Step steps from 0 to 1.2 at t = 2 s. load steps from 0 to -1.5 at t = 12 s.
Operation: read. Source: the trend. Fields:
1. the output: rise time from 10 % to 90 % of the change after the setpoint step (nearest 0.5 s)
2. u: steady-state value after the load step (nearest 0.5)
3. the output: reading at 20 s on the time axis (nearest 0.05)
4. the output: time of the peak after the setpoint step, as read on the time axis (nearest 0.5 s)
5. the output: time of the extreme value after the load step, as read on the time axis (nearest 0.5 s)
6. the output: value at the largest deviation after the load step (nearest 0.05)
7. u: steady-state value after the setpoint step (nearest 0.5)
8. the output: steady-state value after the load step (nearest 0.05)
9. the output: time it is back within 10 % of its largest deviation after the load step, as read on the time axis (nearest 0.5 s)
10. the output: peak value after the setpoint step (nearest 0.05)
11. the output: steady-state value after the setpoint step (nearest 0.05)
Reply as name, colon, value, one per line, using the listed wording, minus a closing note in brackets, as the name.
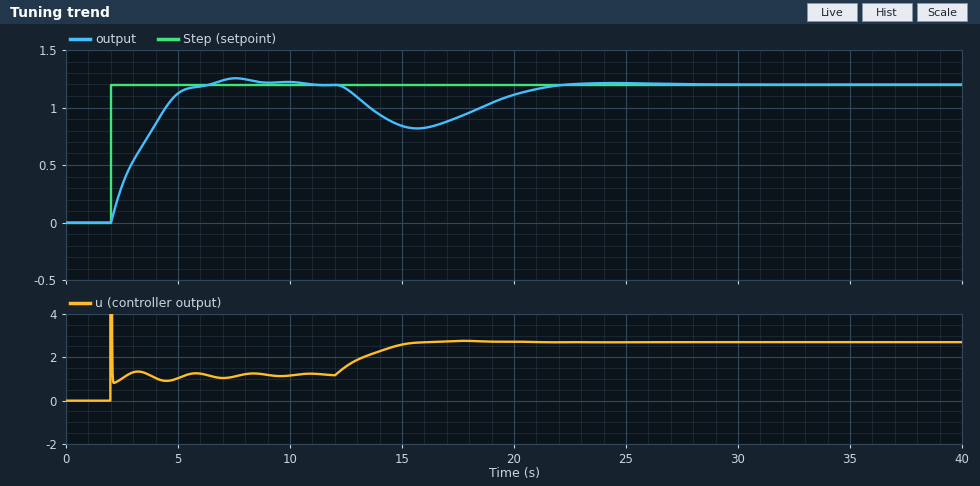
the output: rise time from 10 % to 90 % of the change after the setpoint step: 2.5 s
u: steady-state value after the load step: 2.5
the output: reading at 20 s on the time axis: 1.10
the output: time of the peak after the setpoint step, as read on the time axis: 7.5 s
the output: time of the extreme value after the load step, as read on the time axis: 15.5 s
the output: value at the largest deviation after the load step: 0.80
u: steady-state value after the setpoint step: 1.0
the output: steady-state value after the load step: 1.20
the output: time it is back within 10 % of its largest deviation after the load step, as read on the time axis: 21.0 s
the output: peak value after the setpoint step: 1.25
the output: steady-state value after the setpoint step: 1.20
